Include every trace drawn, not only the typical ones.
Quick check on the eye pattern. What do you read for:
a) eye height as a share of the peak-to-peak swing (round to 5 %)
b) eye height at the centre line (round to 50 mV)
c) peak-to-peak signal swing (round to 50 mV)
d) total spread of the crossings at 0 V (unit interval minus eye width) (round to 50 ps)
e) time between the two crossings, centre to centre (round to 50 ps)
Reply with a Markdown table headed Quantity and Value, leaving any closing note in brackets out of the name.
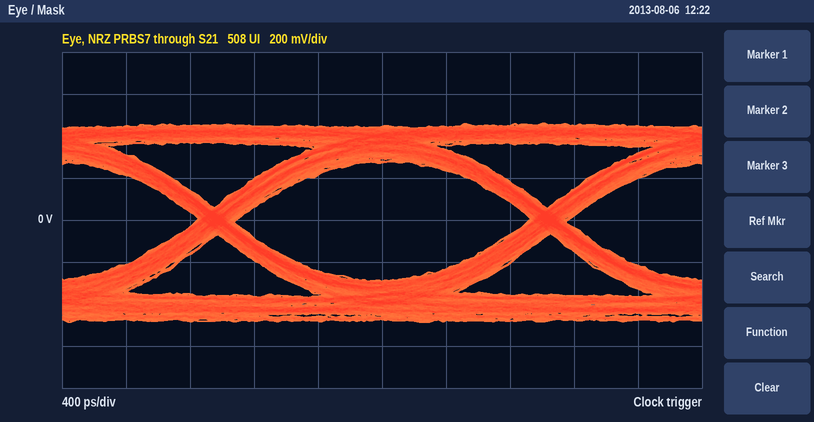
| Quantity | Value |
|---|---|
| eye height as a share of the peak-to-peak swing | 60 % |
| eye height at the centre line | 550 mV |
| peak-to-peak signal swing | 950 mV |
| total spread of the crossings at 0 V (unit interval minus eye width) | 250 ps |
| time between the two crossings, centre to centre | 2.10 ns |
